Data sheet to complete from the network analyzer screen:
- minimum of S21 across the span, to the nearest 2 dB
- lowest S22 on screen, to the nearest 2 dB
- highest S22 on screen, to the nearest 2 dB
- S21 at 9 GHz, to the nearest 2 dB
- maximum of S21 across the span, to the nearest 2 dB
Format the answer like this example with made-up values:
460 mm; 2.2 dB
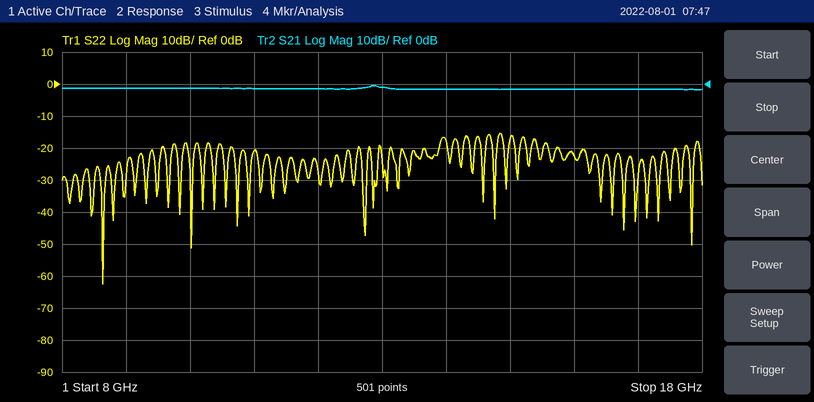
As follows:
-2 dB; -62 dB; -16 dB; -2 dB; 0 dB
